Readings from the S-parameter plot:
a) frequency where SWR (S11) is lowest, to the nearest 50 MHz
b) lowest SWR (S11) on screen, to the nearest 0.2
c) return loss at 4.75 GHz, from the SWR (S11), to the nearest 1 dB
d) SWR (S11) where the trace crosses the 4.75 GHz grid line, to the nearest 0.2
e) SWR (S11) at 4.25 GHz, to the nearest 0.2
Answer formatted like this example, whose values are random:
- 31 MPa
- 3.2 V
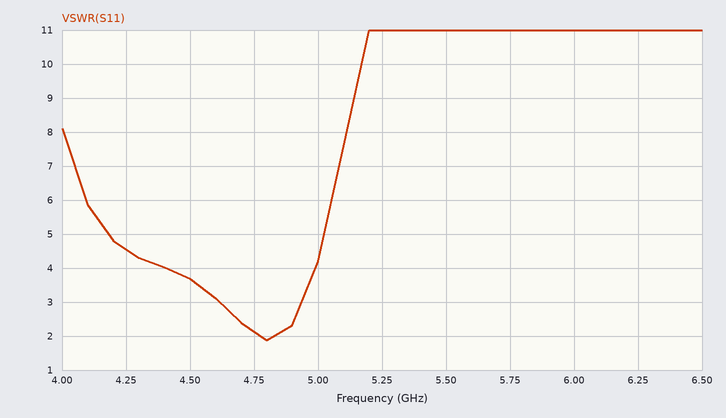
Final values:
- 4.80 GHz
- 1.8
- 9 dB
- 2.2
- 4.6
